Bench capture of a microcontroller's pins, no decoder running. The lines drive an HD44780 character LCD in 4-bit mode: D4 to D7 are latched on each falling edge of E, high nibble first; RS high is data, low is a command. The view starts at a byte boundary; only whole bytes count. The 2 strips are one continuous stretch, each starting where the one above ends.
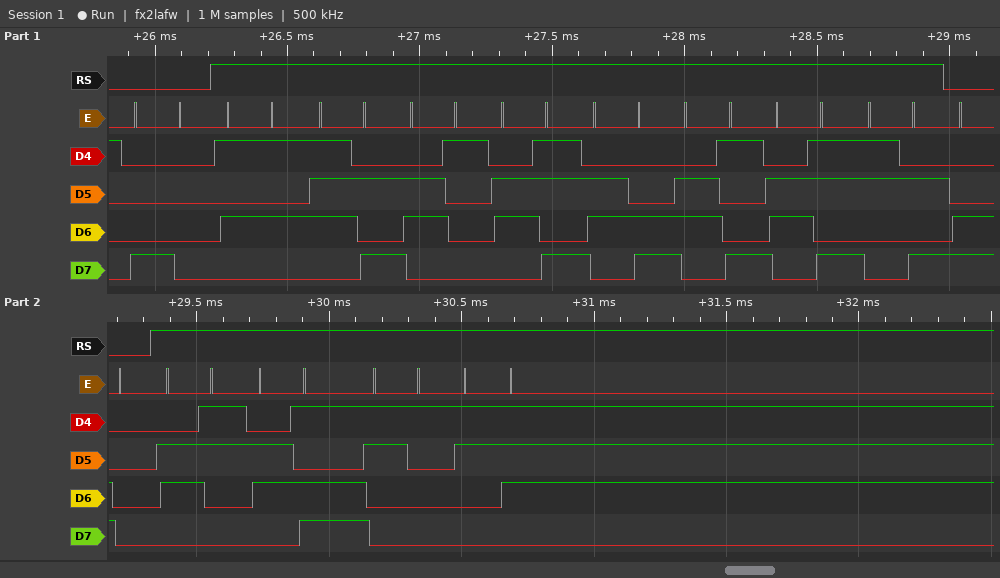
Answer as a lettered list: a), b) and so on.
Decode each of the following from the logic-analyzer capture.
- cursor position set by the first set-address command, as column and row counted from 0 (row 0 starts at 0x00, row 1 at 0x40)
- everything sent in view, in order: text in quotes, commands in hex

a) column 0, row 0
b) 0x80 "Uzaklik:" 0xC0 "cm17"
